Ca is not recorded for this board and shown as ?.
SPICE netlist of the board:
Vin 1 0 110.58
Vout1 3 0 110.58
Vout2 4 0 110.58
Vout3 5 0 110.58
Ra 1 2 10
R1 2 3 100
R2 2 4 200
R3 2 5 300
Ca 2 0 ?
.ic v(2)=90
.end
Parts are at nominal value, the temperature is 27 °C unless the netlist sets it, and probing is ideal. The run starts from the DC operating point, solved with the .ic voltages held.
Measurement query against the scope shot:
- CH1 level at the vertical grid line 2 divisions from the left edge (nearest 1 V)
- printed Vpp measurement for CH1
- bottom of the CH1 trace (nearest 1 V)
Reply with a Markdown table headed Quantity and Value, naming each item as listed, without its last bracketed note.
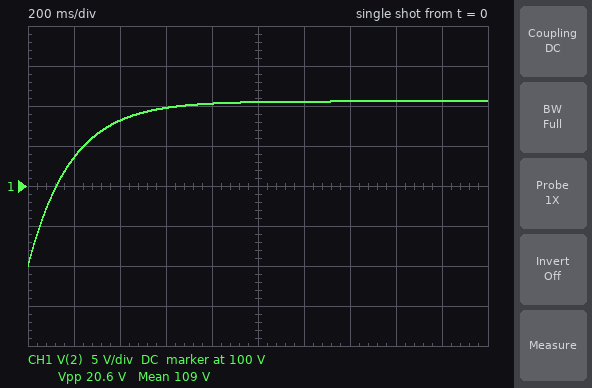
| Quantity | Value |
|---|---|
| CH1 level at the vertical grid line 2 divisions from the left edge | 108 V |
| printed Vpp measurement for CH1 | 20.6 V |
| bottom of the CH1 trace | 90 V |
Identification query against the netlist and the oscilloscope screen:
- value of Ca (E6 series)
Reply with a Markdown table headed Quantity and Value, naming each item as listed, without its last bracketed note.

| Quantity | Value |
|---|---|
| value of Ca | 22 mF |
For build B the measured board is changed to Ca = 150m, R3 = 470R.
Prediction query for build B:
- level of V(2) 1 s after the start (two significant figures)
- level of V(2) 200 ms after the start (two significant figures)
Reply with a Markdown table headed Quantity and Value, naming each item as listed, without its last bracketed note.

| Quantity | Value |
|---|---|
| level of V(2) 1 s after the start | 100 V |
| level of V(2) 200 ms after the start | 93 V |
